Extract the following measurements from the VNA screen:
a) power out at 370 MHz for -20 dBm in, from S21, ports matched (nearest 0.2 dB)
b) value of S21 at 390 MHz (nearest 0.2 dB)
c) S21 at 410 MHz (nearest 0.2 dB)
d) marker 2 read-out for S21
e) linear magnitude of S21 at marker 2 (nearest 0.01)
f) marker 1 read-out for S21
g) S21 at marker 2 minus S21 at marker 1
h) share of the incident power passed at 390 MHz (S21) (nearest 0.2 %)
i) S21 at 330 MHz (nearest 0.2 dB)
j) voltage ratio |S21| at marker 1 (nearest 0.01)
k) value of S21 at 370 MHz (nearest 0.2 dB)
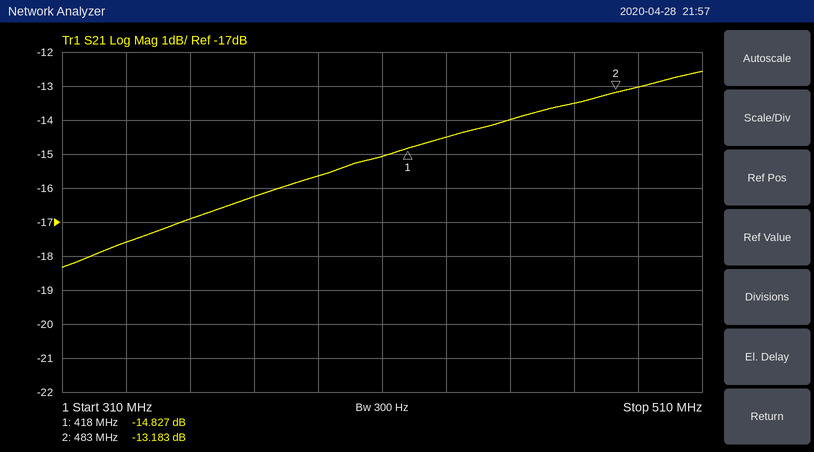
-36.2 dBm
-15.6 dB
-15.0 dB
-13.183 dB
0.22
-14.827 dB
1.644 dB
2.8 %
-17.6 dB
0.18
-16.2 dB
